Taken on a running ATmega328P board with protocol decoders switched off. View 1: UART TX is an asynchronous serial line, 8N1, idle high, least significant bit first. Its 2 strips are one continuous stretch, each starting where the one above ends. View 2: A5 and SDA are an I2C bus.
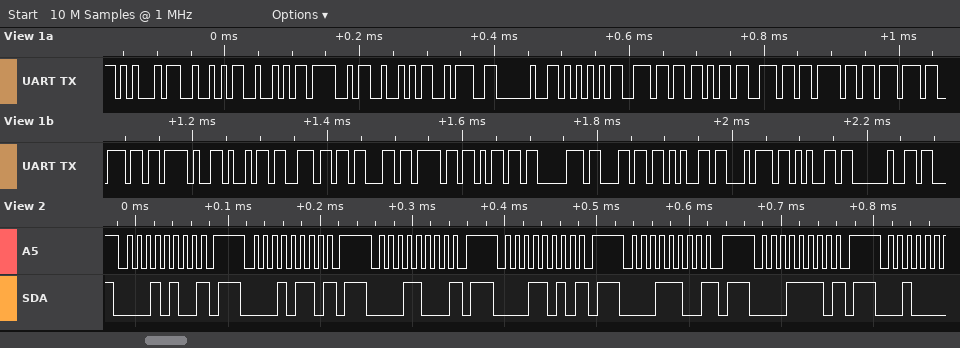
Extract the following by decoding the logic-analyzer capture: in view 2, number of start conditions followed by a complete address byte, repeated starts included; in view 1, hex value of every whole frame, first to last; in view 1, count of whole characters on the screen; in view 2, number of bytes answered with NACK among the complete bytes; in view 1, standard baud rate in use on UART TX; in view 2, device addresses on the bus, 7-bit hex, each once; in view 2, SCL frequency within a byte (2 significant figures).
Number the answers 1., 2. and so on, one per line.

1. 6
2. 45 52 52 4F 52 3A 20 55 6E 6B 6E 6F 77 6E 2F 69 6E 63 6F 6D 70 6C 65 74 65 20
3. 26
4. 6
5. 115200 baud
6. 0x0A 0x0B 0x0C 0x0D 0x0E 0x0F
7. 100 kHz
